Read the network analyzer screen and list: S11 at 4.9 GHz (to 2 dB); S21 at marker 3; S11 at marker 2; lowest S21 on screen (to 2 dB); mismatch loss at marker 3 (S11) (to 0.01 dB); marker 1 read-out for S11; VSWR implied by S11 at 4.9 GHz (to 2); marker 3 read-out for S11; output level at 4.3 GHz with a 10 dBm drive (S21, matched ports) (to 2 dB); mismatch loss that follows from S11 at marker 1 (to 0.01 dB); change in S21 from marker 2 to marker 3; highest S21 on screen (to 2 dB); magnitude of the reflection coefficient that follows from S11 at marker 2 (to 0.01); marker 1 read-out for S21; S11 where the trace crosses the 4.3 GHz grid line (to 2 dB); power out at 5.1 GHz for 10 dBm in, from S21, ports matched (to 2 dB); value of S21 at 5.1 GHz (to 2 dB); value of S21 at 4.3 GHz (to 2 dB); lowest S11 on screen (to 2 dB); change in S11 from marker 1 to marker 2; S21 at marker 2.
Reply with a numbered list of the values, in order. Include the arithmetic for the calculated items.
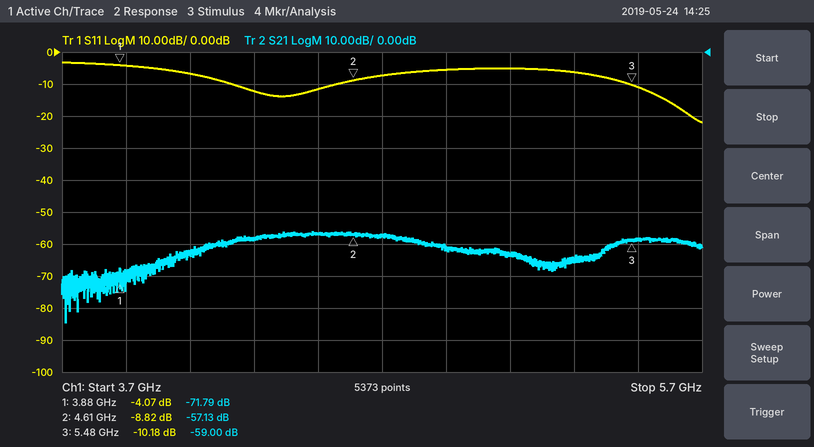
1. -6 dB
2. -59.00 dB
3. -8.82 dB
4. -84 dB
5. −10 log10(1 − 10^(-10.18/10)) ≈ 0.44 dB
6. -4.07 dB
7. |Γ| = 10^(-6/20) = 0.5012; VSWR = (1 + 0.5012)/(1 − 0.5012) ≈ 3.01, so 4 to the nearest 2
8. -10.18 dB
9. 10 dBm + (-58 dB) = -48 dBm
10. −10 log10(1 − 10^(-4.07/10)) ≈ 2.16 dB
11. -59 − (-57.13) = -1.87 dB
12. -56 dB
13. 10^(-8.82/20) ≈ 0.36
14. -71.79 dB
15. -12 dB
16. 10 dBm + (-64 dB) = -54 dBm
17. -64 dB
18. -58 dB
19. -22 dB
20. -8.82 − (-4.07) = -4.75 dB
21. -57.13 dB
